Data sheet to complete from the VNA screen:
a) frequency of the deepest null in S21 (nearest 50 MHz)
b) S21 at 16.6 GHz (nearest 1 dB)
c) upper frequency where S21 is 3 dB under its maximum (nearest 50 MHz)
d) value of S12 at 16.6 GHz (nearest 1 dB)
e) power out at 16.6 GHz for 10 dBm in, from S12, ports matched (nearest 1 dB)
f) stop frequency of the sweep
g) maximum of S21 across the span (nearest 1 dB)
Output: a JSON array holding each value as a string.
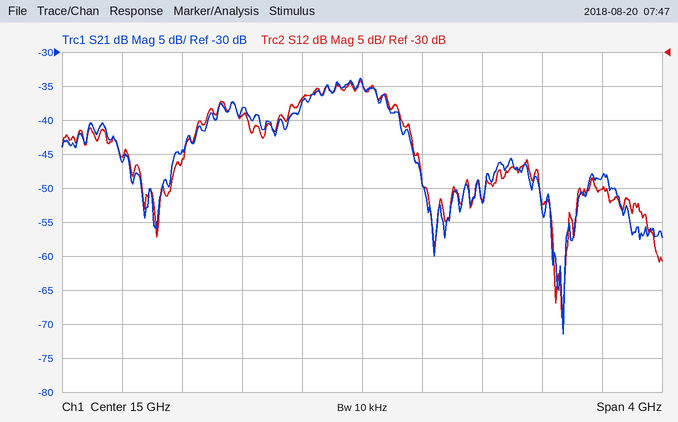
["16.35 GHz", "-48 dB", "15.10 GHz", "-50 dB", "-40 dBm", "17 GHz", "-34 dB"]
